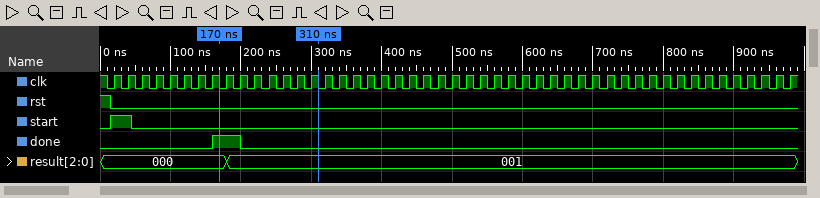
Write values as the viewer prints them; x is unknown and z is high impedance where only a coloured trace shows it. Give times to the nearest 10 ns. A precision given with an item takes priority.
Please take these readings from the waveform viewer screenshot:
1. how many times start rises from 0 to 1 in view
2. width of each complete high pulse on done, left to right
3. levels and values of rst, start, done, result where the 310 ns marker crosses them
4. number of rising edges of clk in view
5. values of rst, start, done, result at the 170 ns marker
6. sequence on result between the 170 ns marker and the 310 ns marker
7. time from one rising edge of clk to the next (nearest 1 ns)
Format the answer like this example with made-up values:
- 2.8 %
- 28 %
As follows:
- 1
- 40 ns
- rst=0, start=0, done=0, result=001
- 49
- rst=0, start=0, done=1, result=000
- 000, 001
- 20 ns
